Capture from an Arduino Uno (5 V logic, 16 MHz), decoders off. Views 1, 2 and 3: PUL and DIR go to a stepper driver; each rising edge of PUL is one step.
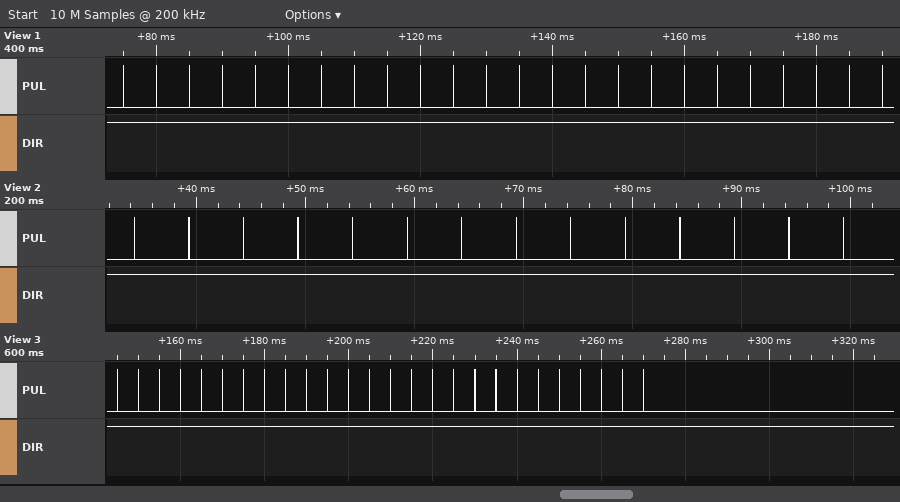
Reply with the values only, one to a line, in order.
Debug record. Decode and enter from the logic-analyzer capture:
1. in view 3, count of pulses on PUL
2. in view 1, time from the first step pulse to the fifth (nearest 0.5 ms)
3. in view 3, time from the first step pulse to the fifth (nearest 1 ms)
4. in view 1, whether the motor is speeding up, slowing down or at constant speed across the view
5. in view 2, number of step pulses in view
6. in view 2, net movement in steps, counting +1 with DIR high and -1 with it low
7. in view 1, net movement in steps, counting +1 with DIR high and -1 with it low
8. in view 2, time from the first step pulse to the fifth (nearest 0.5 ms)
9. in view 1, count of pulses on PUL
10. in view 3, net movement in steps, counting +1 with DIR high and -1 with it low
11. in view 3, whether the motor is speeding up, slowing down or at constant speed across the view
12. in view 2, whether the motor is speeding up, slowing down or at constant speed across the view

26
20.0 ms
20 ms
constant speed
14
+14
+24
20.0 ms
24
+26
constant speed
constant speed
